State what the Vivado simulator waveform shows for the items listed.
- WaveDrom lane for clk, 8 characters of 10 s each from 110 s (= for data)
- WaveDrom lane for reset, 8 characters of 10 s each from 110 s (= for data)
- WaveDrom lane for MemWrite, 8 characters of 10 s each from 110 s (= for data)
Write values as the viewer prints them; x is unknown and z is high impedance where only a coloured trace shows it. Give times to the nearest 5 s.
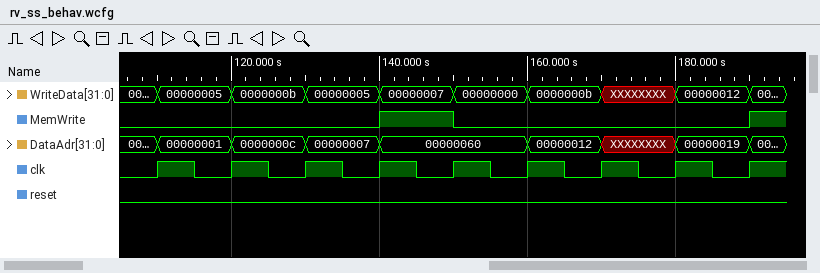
{name: 'clk', wave: 'p.......'}
{name: 'reset', wave: '0.......'}
{name: 'MemWrite', wave: '0..10...'}
